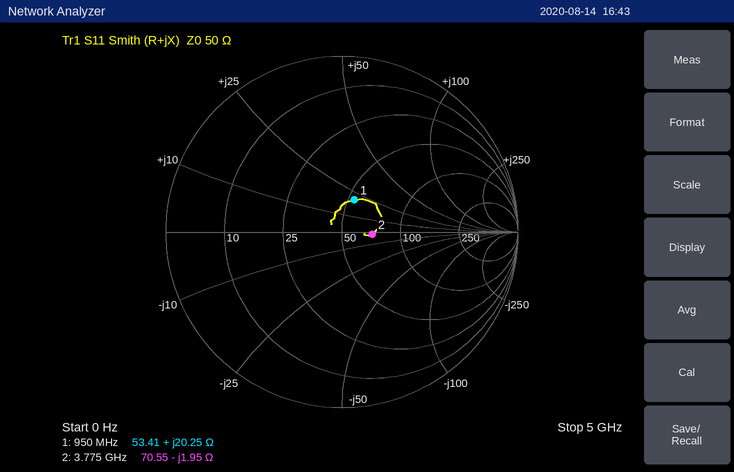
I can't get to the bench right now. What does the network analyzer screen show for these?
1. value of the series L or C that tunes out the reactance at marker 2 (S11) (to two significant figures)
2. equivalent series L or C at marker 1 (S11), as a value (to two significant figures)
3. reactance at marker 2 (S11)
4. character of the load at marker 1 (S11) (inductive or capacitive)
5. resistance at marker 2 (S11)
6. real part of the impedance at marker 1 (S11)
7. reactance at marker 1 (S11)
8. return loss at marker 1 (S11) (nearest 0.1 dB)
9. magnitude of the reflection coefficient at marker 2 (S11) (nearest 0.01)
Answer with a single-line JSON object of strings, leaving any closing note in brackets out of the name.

{"value of the series L or C that tunes out the reactance at marker 2 (S11)": "82 pH", "equivalent series L or C at marker 1 (S11), as a value": "3.4 nH", "reactance at marker 2": "-1.95 Ω", "character of the load at marker 1 (S11)": "inductive", "resistance at marker 2": "70.55 Ω", "real part of the impedance at marker 1": "53.41 Ω", "reactance at marker 1": "+20.25 Ω", "return loss at marker 1 (S11)": "14.2 dB", "magnitude of the reflection coefficient at marker 2 (S11)": "0.17"}
